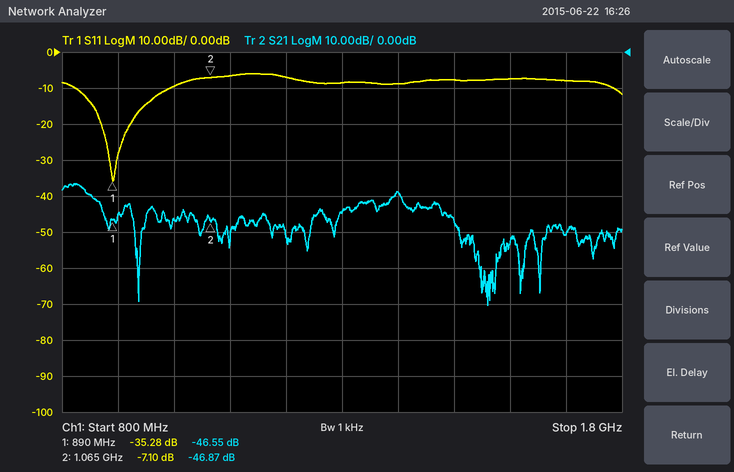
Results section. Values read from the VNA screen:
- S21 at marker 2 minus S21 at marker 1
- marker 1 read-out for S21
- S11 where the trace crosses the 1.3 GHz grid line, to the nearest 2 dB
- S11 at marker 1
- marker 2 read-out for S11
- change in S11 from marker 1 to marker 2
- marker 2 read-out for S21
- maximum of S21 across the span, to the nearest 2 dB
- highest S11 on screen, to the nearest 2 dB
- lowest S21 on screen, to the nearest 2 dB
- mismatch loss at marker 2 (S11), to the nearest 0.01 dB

-0.32 dB
-46.55 dB
-8 dB
-35.28 dB
-7.10 dB
28.18 dB
-46.87 dB
-36 dB
-6 dB
-70 dB
0.94 dB
